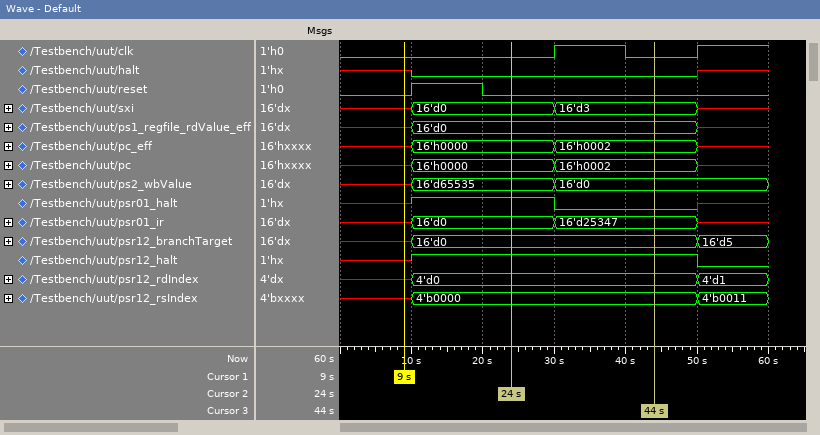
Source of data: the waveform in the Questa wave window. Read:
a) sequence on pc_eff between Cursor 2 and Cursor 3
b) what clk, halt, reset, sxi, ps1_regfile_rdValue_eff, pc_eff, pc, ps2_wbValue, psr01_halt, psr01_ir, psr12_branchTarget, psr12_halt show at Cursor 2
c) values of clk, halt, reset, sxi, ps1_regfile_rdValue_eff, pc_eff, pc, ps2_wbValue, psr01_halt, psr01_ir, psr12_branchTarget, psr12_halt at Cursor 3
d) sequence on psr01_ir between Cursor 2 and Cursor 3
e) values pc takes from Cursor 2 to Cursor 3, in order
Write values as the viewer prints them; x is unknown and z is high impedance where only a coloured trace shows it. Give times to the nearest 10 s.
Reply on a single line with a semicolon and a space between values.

16'h0000, 16'h0002; clk=0, halt=0, reset=0, sxi=16'd0, ps1_regfile_rdValue_eff=16'd0, pc_eff=16'h0000, pc=16'h0000, ps2_wbValue=16'd65535, psr01_halt=1, psr01_ir=16'd0, psr12_branchTarget=16'd0, psr12_halt=1; clk=0, halt=0, reset=0, sxi=16'd3, ps1_regfile_rdValue_eff=16'd0, pc_eff=16'h0002, pc=16'h0002, ps2_wbValue=16'd0, psr01_halt=0, psr01_ir=16'd25347, psr12_branchTarget=16'd0, psr12_halt=1; 16'd0, 16'd25347; 16'h0000, 16'h0002
